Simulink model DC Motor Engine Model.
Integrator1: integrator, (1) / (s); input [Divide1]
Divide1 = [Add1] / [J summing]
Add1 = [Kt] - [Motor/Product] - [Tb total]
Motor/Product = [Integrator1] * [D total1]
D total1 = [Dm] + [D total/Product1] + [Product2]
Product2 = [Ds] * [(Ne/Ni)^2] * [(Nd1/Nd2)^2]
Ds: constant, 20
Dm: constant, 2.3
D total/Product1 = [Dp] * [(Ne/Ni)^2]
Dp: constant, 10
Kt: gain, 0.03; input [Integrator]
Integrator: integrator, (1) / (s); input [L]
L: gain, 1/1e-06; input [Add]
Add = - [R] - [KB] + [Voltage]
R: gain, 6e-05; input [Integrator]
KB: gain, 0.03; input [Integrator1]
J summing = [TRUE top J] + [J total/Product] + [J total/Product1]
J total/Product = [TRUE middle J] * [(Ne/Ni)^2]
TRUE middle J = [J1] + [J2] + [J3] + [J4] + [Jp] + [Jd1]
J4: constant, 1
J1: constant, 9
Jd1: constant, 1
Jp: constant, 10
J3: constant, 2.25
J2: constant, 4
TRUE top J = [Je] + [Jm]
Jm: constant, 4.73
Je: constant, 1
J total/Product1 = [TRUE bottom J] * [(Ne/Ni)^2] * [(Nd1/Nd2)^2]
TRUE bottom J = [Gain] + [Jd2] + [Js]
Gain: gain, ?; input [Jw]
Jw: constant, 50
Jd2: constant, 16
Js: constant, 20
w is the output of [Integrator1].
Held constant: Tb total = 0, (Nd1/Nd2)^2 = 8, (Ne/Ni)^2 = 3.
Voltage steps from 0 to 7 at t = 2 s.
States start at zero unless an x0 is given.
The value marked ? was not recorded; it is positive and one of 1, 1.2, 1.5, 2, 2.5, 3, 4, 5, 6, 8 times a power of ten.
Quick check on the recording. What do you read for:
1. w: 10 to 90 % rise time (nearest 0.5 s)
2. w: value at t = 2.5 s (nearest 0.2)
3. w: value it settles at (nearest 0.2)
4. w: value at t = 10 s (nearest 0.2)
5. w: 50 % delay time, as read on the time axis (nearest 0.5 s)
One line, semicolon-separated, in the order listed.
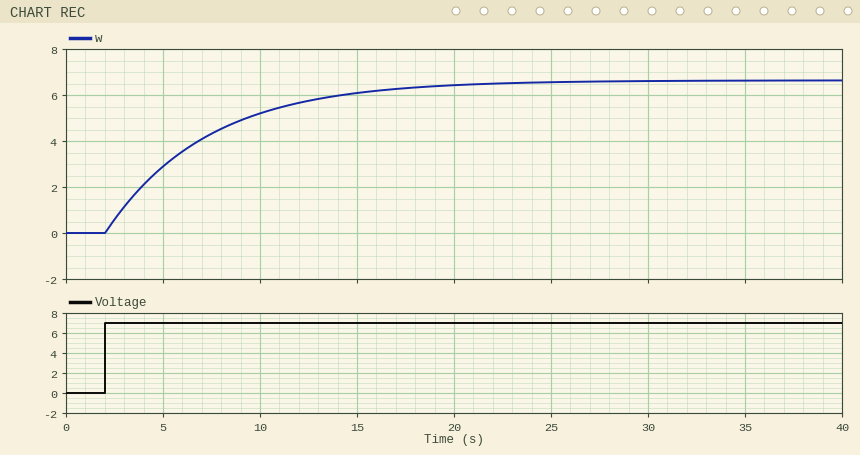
11.5 s; 0.6; 6.6; 5.2; 5.5 s
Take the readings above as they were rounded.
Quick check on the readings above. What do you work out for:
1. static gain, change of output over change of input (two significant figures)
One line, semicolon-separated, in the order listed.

0.94
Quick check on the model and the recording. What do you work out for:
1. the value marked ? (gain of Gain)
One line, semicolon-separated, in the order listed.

1.5
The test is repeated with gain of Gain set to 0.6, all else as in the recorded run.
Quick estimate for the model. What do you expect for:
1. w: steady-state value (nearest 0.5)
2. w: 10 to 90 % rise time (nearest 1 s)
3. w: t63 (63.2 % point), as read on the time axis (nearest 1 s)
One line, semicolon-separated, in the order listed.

6.5; 7 s; 5 s
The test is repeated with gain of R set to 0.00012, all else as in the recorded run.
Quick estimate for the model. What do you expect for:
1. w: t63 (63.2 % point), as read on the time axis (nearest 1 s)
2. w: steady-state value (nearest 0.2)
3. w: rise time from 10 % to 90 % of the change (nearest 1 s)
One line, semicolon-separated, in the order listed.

7 s; 3.4; 12 s
